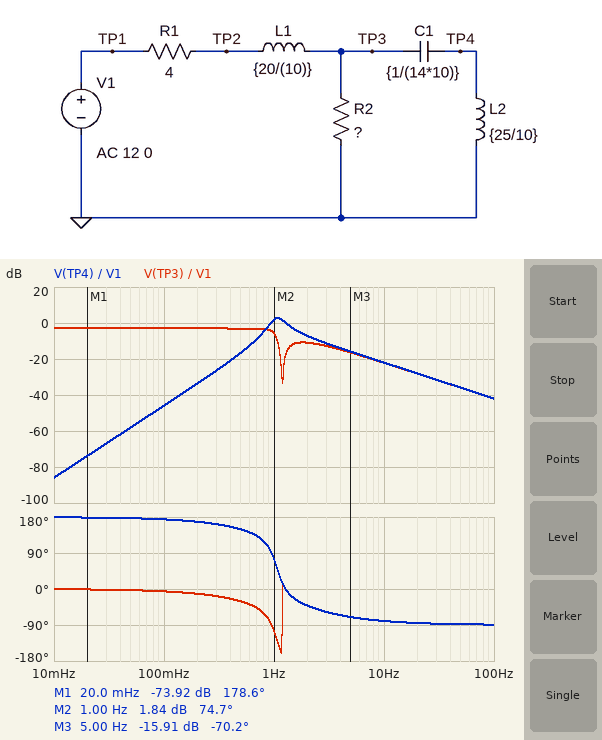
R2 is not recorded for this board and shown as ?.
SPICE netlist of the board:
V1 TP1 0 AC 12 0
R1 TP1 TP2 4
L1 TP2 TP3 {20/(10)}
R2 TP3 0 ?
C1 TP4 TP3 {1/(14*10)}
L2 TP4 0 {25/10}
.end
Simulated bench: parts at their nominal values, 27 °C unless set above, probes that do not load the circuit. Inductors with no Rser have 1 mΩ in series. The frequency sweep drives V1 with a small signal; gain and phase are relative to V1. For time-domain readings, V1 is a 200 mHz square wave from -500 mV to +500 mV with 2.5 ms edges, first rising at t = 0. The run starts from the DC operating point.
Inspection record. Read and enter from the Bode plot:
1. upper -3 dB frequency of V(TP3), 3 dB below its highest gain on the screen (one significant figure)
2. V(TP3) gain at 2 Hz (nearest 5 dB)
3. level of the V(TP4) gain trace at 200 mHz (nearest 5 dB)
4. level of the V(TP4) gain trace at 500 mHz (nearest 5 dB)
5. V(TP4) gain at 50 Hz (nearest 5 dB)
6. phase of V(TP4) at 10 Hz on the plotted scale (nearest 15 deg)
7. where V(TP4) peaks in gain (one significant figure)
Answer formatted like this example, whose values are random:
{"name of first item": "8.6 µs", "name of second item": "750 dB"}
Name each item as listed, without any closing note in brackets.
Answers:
{"upper -3 dB frequency of V(TP3), 3 dB below its highest gain on the screen": "1 Hz", "V(TP3) gain at 2 Hz": "-10 dB", "level of the V(TP4) gain trace at 200 mHz": "-35 dB", "level of the V(TP4) gain trace at 500 mHz": "-15 dB", "V(TP4) gain at 50 Hz": "-35 dB", "phase of V(TP4) at 10 Hz on the plotted scale": "-75 deg", "where V(TP4) peaks in gain": "1 Hz"}
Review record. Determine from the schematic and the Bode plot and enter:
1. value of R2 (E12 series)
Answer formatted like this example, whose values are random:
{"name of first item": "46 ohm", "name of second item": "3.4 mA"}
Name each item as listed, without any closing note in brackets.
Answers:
{"value of R2": "10 Ω"}
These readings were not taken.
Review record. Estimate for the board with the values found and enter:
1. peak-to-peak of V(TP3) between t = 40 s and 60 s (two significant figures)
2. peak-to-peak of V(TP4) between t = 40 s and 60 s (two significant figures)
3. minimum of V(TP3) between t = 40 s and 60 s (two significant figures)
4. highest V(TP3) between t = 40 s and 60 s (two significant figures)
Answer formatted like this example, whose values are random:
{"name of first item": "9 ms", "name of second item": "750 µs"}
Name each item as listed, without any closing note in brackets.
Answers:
{"peak-to-peak of V(TP3) between t = 40 s and 60 s": "930 mV", "peak-to-peak of V(TP4) between t = 40 s and 60 s": "590 mV", "minimum of V(TP3) between t = 40 s and 60 s": "-460 mV", "highest V(TP3) between t = 40 s and 60 s": "460 mV"}
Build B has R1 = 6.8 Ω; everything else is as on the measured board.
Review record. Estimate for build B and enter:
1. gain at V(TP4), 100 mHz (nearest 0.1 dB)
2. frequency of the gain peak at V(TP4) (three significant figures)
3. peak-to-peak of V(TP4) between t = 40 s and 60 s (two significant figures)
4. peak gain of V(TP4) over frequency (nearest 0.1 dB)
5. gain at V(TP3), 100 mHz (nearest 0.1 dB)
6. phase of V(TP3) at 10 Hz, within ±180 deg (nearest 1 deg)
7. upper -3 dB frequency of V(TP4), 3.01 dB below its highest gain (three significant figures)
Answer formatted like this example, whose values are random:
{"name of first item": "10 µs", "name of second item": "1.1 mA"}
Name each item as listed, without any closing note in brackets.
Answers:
{"gain at V(TP4), 100 mHz": "-47.5 dB", "frequency of the gain peak at V(TP4)": "1.11 Hz", "peak-to-peak of V(TP4) between t = 40 s and 60 s": "520 mV", "peak gain of V(TP4) over frequency": "1.8 dB", "gain at V(TP3), 100 mHz": "-4.5 dB", "phase of V(TP3) at 10 Hz, within ±180 deg": "-79 deg", "upper -3 dB frequency of V(TP4), 3.01 dB below its highest gain": "1.34 Hz"}
